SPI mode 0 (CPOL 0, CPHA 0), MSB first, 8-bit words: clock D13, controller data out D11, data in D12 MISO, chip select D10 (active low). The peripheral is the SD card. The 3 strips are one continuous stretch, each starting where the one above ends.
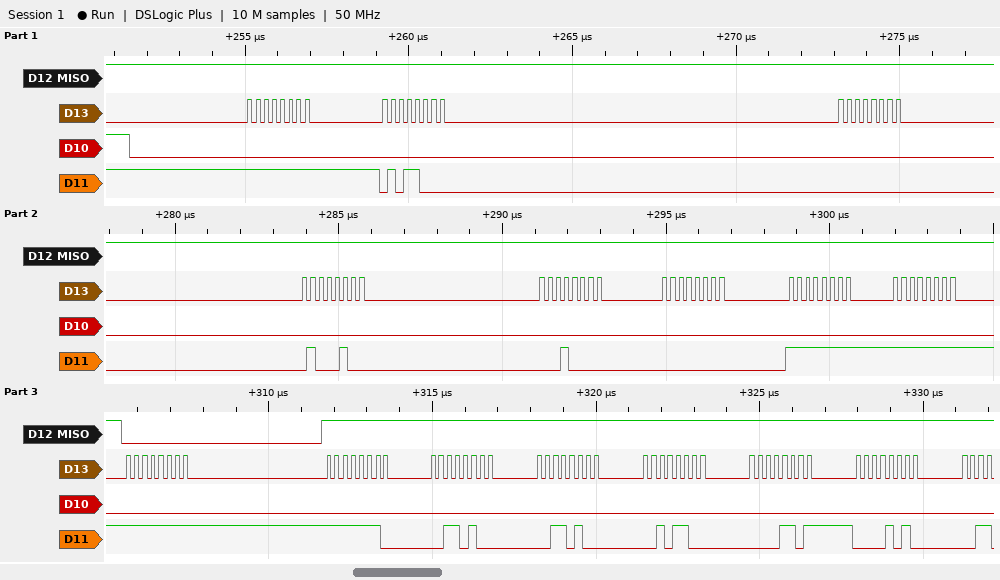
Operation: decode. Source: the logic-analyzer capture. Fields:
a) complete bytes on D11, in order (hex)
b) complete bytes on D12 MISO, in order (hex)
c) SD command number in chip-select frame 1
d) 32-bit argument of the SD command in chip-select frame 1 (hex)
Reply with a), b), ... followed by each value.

a) 0xFF 0x58 0x00 0x44 0x10 0x00 0xFF 0xFF 0xFF 0xFE 0x34 0x34 0x2C 0x0D 0x0A
b) 0xFF 0xFF 0xFF 0xFF 0xFF 0xFF 0xFF 0xFF 0x00 0xFF 0xFF 0xFF 0xFF 0xFF 0xFF
c) CMD24
d) 0x00441000
